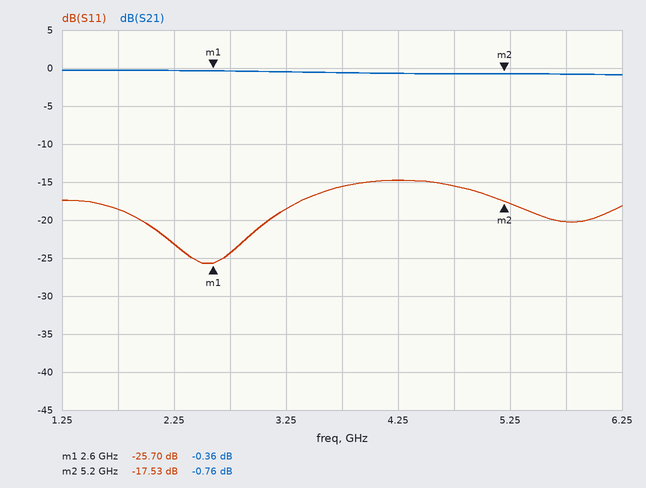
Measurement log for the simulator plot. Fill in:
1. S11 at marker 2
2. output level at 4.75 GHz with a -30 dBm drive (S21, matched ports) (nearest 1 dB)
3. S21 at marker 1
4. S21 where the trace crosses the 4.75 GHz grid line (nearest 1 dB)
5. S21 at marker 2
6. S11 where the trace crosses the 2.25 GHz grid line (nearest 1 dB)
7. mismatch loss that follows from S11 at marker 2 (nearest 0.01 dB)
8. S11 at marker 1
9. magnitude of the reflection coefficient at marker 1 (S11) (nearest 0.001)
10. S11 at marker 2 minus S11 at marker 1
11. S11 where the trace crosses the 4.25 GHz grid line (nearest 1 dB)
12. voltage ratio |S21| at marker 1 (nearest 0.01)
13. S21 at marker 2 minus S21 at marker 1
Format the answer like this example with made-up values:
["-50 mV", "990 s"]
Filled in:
["-17.53 dB", "-31 dBm", "-0.36 dB", "-1 dB", "-0.76 dB", "-23 dB", "0.08 dB", "-25.70 dB", "0.052", "8.17 dB", "-15 dB", "0.96", "-0.40 dB"]
